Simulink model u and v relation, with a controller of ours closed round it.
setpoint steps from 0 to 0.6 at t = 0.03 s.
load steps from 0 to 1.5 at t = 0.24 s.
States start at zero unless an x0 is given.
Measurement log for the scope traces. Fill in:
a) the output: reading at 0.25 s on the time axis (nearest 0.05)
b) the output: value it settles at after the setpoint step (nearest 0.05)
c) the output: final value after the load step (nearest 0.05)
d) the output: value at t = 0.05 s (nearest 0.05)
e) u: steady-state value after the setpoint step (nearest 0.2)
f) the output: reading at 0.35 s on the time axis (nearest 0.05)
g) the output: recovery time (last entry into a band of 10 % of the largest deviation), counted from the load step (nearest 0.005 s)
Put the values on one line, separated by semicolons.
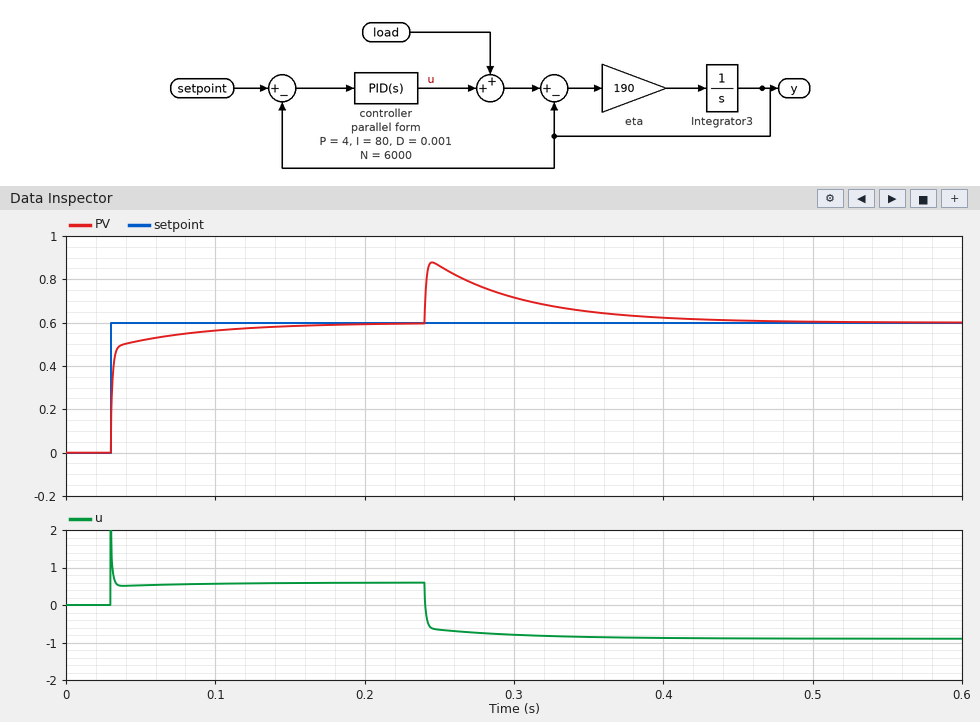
0.85; 0.60; 0.60; 0.50; 0.6; 0.65; 0.145 s
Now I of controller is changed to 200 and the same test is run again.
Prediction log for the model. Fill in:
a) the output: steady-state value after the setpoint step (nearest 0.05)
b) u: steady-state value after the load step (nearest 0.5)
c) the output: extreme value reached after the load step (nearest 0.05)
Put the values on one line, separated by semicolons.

0.60; -1.0; 0.85
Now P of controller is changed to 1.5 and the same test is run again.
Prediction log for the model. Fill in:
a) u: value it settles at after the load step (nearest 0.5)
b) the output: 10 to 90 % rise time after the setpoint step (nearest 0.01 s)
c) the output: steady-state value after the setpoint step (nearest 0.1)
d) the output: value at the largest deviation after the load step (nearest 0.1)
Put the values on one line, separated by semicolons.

-1.0; 0.04 s; 0.6; 1.1
